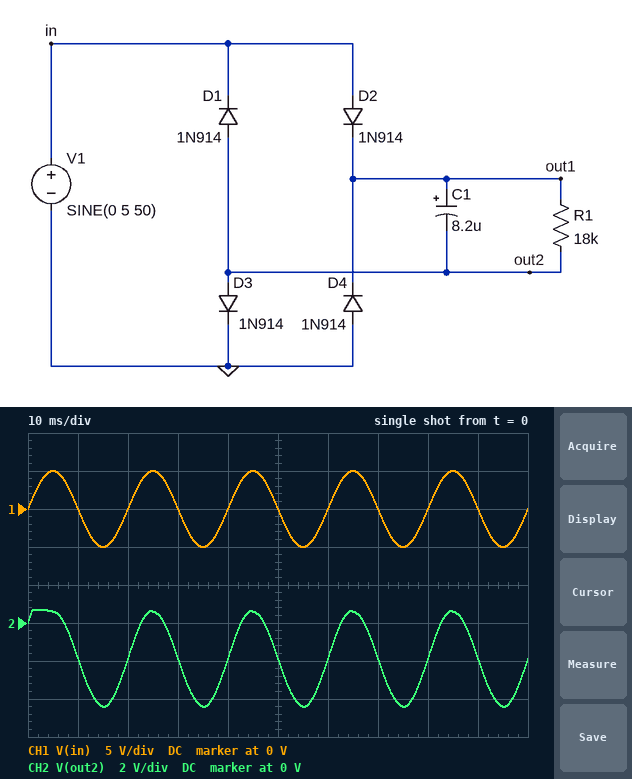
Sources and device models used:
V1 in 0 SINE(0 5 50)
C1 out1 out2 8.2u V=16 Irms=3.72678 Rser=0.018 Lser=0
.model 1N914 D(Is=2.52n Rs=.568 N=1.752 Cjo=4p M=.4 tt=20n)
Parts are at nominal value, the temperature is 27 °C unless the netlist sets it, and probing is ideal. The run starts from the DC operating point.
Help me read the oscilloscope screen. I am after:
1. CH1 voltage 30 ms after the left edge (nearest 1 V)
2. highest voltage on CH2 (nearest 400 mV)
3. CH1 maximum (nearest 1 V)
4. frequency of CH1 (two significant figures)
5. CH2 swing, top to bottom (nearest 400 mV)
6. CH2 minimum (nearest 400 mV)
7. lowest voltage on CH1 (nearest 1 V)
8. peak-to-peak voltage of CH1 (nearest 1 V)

0 V
800 mV
5 V
50 Hz
5.2 V
-4.4 V
-5 V
10 V
